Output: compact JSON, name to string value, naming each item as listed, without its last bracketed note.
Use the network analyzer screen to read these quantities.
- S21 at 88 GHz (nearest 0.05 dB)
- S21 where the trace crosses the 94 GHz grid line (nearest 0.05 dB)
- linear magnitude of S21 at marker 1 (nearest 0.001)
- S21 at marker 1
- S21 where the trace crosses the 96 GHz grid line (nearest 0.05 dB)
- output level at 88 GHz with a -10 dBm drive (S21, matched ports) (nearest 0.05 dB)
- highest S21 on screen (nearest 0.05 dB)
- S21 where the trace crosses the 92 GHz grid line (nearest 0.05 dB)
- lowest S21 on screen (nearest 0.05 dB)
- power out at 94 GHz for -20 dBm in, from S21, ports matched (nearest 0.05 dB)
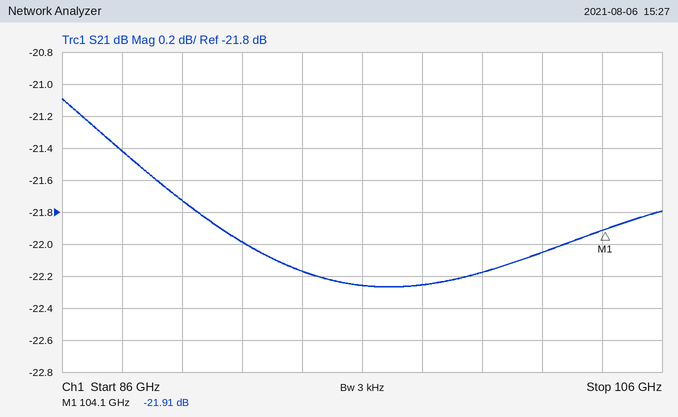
{"S21 at 88 GHz": "-21.40 dB", "S21 where the trace crosses the 94 GHz grid line": "-22.15 dB", "linear magnitude of S21 at marker 1": "0.080", "S21 at marker 1": "-21.91 dB", "S21 where the trace crosses the 96 GHz grid line": "-22.25 dB", "output level at 88 GHz with a -10 dBm drive (S21, matched ports)": "-31.40 dBm", "highest S21 on screen": "-21.10 dB", "S21 where the trace crosses the 92 GHz grid line": "-22.00 dB", "lowest S21 on screen": "-22.25 dB", "power out at 94 GHz for -20 dBm in, from S21, ports matched": "-42.15 dBm"}
